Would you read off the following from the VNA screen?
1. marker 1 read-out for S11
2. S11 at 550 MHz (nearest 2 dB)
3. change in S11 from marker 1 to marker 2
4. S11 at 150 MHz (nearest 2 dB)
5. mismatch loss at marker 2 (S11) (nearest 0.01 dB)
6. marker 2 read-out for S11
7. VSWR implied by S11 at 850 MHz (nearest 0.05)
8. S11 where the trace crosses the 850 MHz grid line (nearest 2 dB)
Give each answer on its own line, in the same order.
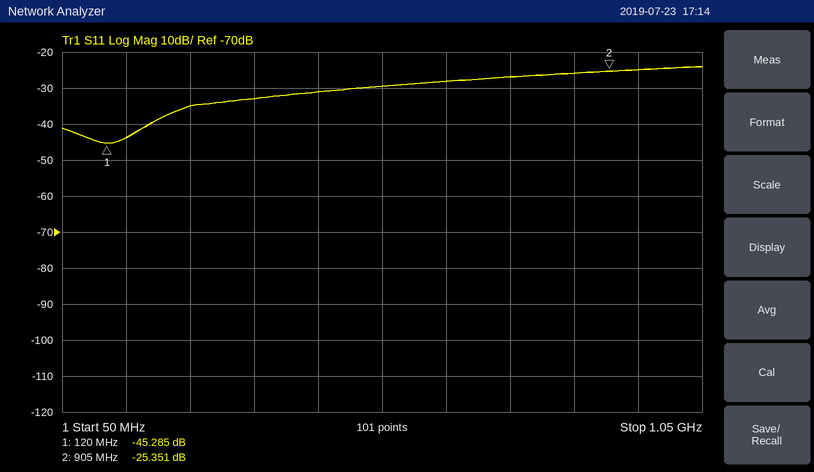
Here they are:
-45.285 dB
-30 dB
19.934 dB
-44 dB
0.01 dB
-25.351 dB
1.10
-26 dB
